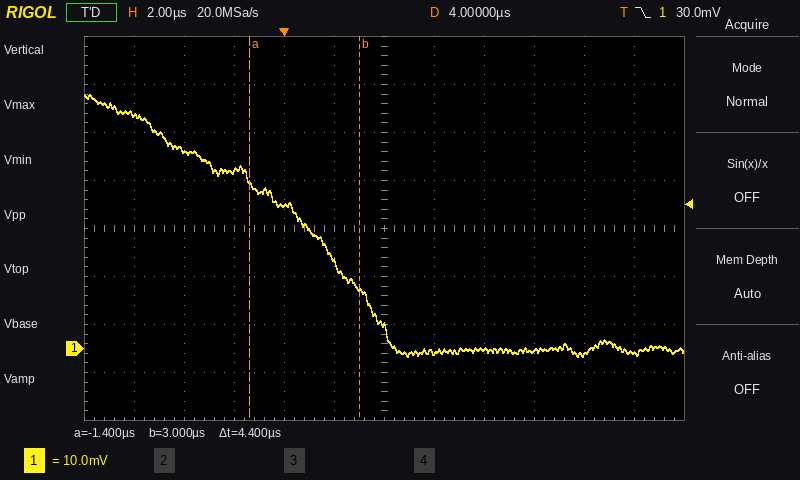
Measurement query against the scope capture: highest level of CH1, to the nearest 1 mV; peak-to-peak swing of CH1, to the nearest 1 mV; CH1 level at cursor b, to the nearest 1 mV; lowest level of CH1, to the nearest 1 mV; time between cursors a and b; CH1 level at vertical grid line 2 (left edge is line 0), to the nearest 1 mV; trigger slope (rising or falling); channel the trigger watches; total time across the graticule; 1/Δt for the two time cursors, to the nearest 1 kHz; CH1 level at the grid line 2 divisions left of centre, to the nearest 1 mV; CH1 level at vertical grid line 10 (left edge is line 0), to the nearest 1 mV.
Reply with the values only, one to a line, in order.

53 mV
55 mV
12 mV
-2 mV
4.4 µs
41 mV
falling
CH1
24 µs
227 kHz
30 mV
-1 mV
